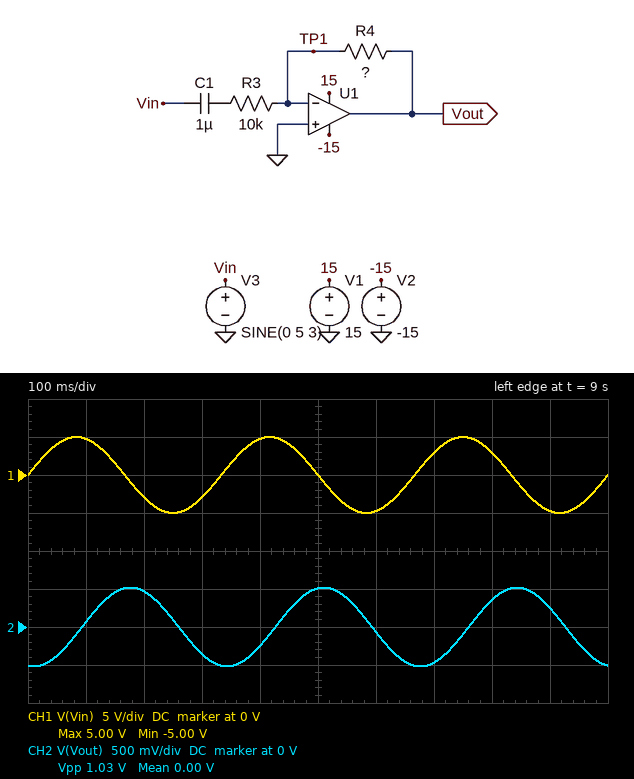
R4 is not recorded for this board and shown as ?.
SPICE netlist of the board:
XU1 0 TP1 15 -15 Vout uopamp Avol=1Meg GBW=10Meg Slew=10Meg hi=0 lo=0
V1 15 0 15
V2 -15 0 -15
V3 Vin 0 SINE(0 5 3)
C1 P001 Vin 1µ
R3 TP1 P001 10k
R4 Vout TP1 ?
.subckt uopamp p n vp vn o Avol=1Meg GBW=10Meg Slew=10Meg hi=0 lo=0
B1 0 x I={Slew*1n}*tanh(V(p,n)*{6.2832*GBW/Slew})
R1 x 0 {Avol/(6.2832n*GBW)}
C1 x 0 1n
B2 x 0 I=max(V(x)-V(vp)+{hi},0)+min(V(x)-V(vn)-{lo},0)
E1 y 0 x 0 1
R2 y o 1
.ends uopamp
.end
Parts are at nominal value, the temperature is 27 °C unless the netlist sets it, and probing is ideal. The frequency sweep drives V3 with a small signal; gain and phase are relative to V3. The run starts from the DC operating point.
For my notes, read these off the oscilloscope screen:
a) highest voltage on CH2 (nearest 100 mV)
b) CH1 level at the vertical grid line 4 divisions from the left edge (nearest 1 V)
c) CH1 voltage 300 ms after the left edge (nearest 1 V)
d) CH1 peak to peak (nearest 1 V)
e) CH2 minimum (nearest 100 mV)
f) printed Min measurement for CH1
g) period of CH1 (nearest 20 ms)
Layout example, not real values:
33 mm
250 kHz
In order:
500 mV
5 V
-3 V
10 V
-500 mV
-5.00 V
340 ms
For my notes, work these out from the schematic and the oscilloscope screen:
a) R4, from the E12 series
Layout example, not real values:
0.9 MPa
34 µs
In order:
5.6 kΩ
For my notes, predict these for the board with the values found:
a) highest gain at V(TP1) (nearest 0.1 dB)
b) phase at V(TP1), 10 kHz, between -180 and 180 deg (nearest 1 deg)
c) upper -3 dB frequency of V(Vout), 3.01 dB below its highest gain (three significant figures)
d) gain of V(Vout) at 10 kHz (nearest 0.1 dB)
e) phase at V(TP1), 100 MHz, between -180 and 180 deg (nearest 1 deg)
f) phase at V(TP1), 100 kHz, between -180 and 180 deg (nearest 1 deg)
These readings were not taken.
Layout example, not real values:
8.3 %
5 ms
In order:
-8.9 dB
90 deg
6.41 MHz
-5.0 dB
4 deg
89 deg
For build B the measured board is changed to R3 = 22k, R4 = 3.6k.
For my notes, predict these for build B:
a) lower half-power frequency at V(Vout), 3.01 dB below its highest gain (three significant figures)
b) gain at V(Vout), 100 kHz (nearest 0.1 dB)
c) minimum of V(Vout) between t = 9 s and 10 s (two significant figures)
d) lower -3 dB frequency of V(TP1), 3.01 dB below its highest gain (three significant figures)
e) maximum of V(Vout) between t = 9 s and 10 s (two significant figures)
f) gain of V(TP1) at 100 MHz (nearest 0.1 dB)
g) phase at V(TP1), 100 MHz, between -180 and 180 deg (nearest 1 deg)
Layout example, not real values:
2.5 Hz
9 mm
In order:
7.23 Hz
-15.7 dB
-310 mV
8.59 MHz
310 mV
-17.1 dB
5 deg
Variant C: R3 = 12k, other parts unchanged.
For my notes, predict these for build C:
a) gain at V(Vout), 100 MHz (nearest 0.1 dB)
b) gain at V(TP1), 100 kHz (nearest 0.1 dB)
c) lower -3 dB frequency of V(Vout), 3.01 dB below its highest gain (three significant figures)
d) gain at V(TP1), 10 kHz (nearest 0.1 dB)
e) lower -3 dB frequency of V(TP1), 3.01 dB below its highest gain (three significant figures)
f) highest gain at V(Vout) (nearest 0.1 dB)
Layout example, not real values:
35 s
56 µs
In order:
-30.0 dB
-46.6 dB
13.3 Hz
-66.6 dB
6.82 MHz
-6.6 dB
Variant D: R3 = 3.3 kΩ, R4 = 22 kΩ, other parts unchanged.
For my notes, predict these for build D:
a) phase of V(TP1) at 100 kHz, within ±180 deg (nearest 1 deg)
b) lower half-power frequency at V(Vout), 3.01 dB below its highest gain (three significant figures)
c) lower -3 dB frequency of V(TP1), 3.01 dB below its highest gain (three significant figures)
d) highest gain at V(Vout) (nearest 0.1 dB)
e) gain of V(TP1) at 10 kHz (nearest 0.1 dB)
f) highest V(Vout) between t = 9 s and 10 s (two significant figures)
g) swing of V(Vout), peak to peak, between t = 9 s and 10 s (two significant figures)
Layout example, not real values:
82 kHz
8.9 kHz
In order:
86 deg
48.2 Hz
1.30 MHz
16.5 dB
-43.5 dB
2.1 V
4.1 V
